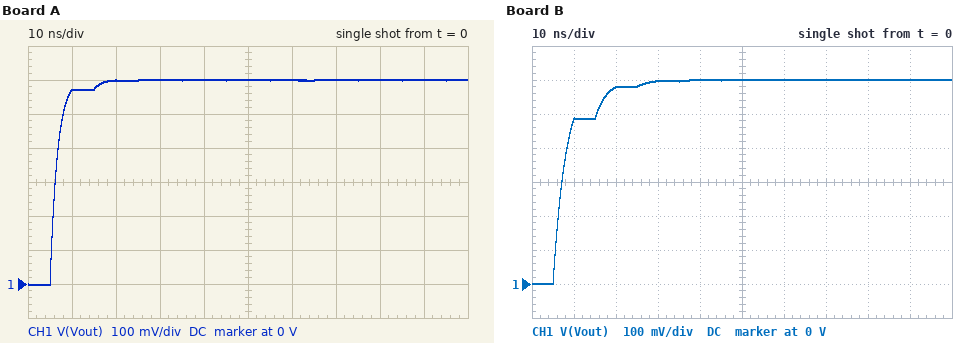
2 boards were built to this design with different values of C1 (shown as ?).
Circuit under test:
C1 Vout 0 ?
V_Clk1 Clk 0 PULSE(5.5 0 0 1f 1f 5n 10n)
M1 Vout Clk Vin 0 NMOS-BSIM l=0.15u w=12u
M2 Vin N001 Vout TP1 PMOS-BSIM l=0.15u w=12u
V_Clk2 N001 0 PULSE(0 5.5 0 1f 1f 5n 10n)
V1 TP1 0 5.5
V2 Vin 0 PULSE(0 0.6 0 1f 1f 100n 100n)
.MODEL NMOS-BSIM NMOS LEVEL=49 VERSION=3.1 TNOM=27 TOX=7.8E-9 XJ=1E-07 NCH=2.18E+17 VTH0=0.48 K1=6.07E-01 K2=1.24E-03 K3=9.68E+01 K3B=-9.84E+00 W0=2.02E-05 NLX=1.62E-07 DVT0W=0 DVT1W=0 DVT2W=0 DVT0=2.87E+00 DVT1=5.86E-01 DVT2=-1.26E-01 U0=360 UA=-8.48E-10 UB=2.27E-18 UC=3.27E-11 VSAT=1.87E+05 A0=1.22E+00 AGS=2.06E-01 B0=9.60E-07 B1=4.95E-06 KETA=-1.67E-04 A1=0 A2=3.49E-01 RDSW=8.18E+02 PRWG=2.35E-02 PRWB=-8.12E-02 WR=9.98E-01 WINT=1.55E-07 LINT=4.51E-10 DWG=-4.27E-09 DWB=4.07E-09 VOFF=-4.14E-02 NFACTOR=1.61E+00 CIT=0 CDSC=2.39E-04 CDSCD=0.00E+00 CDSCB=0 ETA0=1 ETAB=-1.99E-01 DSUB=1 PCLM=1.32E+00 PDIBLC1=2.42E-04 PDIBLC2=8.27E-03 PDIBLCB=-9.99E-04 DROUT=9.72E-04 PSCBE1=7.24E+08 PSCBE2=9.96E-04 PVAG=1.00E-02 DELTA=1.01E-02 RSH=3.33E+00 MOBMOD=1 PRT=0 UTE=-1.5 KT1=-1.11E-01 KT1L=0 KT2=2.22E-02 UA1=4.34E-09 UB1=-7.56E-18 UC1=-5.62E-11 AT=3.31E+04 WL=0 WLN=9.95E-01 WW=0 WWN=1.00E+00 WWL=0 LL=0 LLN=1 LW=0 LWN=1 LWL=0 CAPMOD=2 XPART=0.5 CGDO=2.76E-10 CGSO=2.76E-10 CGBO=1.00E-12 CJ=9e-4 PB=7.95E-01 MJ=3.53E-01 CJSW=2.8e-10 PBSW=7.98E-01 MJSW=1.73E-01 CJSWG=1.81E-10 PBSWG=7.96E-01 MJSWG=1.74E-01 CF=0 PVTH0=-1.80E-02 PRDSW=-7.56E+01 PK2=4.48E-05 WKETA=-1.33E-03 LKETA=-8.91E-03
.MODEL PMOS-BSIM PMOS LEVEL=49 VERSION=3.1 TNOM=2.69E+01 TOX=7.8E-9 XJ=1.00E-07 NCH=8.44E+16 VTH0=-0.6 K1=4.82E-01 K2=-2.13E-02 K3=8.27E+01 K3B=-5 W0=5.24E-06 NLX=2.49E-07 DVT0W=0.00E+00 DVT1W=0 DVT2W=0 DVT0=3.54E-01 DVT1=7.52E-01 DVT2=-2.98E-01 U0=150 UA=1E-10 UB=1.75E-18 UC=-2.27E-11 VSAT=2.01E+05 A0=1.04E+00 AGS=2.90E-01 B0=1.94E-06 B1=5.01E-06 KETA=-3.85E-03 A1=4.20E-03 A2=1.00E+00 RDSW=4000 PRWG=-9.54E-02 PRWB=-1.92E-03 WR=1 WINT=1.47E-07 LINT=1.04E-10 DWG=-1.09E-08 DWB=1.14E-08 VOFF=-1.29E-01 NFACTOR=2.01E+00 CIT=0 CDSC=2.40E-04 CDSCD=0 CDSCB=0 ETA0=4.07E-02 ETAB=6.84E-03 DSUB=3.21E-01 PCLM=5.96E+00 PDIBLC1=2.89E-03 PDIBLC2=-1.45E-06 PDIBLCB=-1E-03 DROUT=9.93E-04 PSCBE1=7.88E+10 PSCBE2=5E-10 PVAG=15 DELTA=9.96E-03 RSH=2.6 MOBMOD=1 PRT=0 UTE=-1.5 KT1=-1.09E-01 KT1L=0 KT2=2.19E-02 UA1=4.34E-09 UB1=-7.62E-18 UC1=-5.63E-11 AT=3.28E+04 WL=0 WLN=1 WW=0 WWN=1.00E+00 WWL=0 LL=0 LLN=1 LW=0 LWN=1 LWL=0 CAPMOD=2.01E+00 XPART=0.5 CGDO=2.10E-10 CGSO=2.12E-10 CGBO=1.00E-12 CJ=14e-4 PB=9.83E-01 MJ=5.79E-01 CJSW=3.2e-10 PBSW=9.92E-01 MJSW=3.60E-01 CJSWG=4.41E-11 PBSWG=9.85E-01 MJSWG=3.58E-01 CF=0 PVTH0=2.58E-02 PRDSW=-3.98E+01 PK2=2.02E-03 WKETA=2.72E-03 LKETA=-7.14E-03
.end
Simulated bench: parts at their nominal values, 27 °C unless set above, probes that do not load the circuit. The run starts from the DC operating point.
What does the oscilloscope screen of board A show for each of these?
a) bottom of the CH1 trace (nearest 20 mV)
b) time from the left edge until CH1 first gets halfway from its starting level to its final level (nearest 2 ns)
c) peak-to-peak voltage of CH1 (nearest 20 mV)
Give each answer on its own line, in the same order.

0 V
6 ns
600 mV
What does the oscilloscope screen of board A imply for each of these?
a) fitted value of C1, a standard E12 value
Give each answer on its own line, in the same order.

15 pF
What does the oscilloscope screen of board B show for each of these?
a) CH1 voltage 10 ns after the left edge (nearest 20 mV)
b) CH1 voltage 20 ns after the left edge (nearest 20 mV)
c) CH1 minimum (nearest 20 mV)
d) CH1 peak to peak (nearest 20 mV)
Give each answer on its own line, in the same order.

480 mV
580 mV
0 V
600 mV
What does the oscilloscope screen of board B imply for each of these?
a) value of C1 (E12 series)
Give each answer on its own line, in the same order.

27 pF
